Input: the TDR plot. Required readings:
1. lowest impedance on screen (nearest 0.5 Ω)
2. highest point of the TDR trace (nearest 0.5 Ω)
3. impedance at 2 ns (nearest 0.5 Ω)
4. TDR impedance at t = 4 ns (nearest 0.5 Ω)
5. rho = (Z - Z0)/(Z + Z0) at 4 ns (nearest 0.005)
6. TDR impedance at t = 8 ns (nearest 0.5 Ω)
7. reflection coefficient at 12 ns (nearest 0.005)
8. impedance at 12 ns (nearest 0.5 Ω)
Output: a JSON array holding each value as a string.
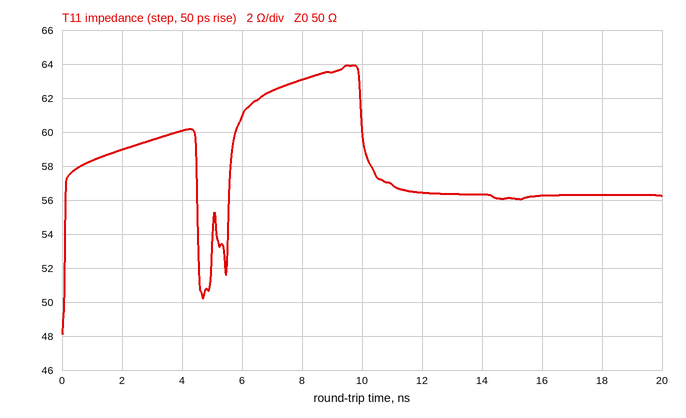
["48.0 Ω", "64.0 Ω", "59.0 Ω", "60.0 Ω", "+0.090", "63.0 Ω", "+0.060", "56.5 Ω"]
